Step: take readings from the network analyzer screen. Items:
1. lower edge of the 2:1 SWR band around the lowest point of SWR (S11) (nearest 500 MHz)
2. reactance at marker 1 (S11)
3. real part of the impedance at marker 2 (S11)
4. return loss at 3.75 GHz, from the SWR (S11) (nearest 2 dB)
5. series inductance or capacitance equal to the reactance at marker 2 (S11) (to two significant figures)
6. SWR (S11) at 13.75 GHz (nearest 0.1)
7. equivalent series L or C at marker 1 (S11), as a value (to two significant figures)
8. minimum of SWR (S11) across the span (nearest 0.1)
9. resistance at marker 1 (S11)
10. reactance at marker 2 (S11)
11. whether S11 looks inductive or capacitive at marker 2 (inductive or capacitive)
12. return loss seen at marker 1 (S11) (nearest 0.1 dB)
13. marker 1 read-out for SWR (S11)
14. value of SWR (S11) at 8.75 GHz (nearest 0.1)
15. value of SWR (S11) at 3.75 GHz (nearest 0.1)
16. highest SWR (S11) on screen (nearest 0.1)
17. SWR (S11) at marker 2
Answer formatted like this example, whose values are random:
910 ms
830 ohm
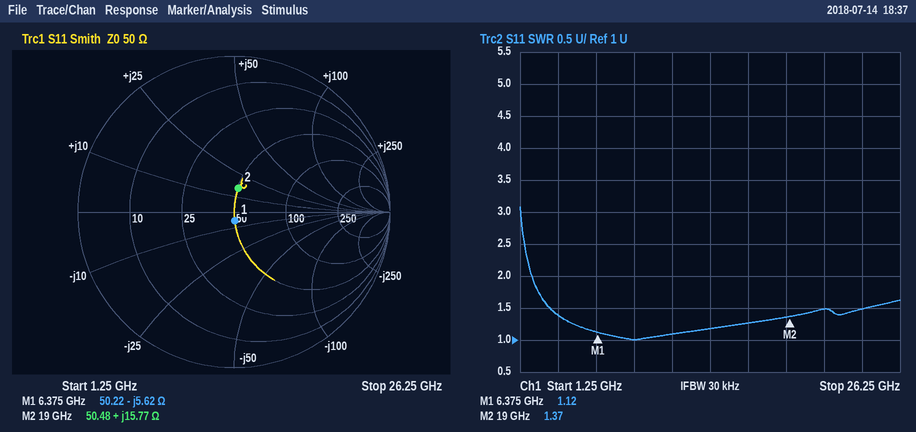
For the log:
2.0 GHz
-5.62 Ω
50.48 Ω
16 dB
130 pH
1.2
4.4 pF
1.0
50.22 Ω
+15.77 Ω
inductive
25.0 dB
1.12
1.0
1.4
3.1
1.37
